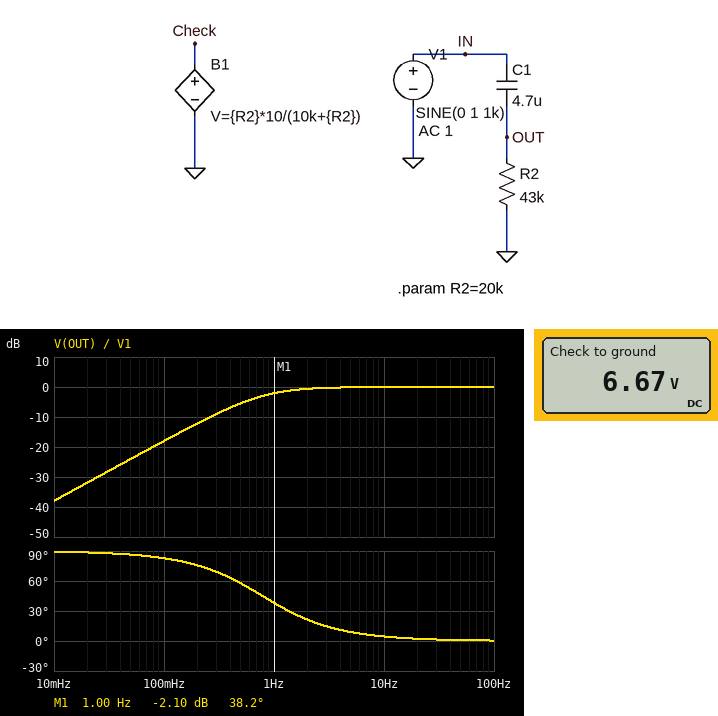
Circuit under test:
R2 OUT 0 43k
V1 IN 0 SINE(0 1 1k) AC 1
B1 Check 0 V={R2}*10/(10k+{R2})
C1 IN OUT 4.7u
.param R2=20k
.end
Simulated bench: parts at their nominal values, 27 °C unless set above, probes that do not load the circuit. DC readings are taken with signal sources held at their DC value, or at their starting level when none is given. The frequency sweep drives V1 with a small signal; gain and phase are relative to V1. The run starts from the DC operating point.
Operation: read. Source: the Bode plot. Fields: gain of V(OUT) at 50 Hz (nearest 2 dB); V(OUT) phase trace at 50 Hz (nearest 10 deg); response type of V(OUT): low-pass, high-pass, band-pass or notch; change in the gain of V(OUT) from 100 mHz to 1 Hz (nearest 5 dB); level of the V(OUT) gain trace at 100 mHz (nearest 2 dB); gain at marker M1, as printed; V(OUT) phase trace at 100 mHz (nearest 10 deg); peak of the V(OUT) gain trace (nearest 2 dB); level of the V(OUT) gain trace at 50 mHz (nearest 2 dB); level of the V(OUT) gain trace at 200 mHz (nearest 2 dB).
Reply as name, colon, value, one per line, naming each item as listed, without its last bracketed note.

gain of V(OUT) at 50 Hz: 0 dB
V(OUT) phase trace at 50 Hz: 0 deg
response type of V(OUT): low-pass, high-pass, band-pass or notch: high-pass
change in the gain of V(OUT) from 100 mHz to 1 Hz: 15 dB
level of the V(OUT) gain trace at 100 mHz: -18 dB
gain at marker M1, as printed: -2.10 dB
V(OUT) phase trace at 100 mHz: 80 deg
peak of the V(OUT) gain trace: 0 dB
level of the V(OUT) gain trace at 50 mHz: -24 dB
level of the V(OUT) gain trace at 200 mHz: -12 dB
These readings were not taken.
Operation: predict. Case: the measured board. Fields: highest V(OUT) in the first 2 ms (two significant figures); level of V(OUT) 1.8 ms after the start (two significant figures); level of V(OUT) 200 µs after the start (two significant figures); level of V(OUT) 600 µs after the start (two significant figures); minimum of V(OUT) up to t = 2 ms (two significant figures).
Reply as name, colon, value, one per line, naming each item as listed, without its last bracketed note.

highest V(OUT) in the first 2 ms: 1.0 V
level of V(OUT) 1.8 ms after the start: -950 mV
level of V(OUT) 200 µs after the start: 950 mV
level of V(OUT) 600 µs after the start: -590 mV
minimum of V(OUT) up to t = 2 ms: -1.0 V
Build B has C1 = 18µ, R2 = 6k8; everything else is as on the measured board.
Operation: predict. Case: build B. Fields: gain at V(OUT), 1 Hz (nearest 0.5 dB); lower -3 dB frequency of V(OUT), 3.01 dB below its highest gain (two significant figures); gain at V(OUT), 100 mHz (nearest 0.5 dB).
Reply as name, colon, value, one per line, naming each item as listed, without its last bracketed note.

gain at V(OUT), 1 Hz: -4.5 dB
lower -3 dB frequency of V(OUT), 3.01 dB below its highest gain: 1.3 Hz
gain at V(OUT), 100 mHz: -22.5 dB
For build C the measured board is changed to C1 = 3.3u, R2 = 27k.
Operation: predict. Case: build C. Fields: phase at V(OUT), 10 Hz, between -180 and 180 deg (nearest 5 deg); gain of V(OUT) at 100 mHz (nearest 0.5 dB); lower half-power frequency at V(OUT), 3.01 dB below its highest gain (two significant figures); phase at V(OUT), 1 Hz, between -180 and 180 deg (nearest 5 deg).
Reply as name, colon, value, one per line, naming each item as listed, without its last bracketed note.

phase at V(OUT), 10 Hz, between -180 and 180 deg: 10 deg
gain of V(OUT) at 100 mHz: -25.0 dB
lower half-power frequency at V(OUT), 3.01 dB below its highest gain: 1.8 Hz
phase at V(OUT), 1 Hz, between -180 and 180 deg: 60 deg
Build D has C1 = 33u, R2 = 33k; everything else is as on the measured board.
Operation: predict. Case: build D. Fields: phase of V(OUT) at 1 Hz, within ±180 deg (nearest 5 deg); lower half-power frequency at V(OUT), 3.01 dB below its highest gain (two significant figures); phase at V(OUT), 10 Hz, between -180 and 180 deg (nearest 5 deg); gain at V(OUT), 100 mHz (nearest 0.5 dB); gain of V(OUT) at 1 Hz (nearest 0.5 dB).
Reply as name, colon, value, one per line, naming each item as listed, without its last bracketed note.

phase of V(OUT) at 1 Hz, within ±180 deg: 10 deg
lower half-power frequency at V(OUT), 3.01 dB below its highest gain: 150 mHz
phase at V(OUT), 10 Hz, between -180 and 180 deg: 0 deg
gain at V(OUT), 100 mHz: -5.0 dB
gain of V(OUT) at 1 Hz: 0 dB
